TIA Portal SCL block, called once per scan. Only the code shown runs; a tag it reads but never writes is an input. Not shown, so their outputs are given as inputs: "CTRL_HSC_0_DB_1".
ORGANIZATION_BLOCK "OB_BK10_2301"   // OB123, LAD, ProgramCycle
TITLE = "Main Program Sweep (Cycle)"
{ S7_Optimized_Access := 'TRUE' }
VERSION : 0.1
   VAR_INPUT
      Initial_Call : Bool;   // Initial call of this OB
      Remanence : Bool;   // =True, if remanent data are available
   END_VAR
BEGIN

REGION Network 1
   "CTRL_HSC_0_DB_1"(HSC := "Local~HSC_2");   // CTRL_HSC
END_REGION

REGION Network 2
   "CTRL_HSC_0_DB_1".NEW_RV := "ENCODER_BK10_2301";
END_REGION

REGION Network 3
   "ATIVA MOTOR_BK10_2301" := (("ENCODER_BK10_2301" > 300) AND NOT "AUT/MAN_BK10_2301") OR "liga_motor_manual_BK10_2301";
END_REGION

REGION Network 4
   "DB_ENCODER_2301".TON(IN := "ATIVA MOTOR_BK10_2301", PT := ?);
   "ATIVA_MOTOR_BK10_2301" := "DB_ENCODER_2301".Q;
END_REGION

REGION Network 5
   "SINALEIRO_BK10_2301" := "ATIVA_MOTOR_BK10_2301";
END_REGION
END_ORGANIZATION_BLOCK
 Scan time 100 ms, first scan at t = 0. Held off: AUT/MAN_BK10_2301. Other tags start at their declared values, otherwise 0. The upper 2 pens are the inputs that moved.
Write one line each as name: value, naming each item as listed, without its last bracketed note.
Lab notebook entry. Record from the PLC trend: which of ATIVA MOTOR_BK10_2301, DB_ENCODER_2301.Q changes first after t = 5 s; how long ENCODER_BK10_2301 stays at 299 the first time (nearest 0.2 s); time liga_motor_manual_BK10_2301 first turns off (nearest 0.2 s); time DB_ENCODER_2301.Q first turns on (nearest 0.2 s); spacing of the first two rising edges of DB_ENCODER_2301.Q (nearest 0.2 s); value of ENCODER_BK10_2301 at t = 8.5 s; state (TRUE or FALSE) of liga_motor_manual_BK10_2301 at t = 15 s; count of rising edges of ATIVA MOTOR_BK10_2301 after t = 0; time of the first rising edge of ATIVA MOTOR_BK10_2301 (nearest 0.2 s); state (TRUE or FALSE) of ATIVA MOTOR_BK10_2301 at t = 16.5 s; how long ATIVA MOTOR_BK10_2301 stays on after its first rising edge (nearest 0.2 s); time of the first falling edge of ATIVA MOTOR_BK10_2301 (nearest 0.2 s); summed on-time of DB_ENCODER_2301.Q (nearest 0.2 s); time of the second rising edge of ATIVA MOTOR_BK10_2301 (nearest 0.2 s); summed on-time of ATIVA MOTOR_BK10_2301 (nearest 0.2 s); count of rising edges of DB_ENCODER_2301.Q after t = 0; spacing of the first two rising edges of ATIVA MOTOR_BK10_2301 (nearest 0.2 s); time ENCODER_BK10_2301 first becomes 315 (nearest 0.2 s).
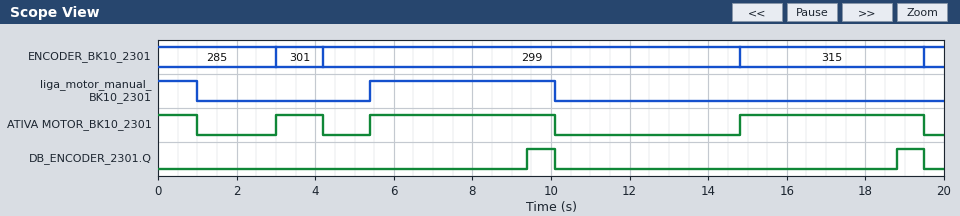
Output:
which of ATIVA MOTOR_BK10_2301, DB_ENCODER_2301.Q changes first after t = 5 s: ATIVA MOTOR_BK10_2301
how long ENCODER_BK10_2301 stays at 299 the first time: 10.6 s
time liga_motor_manual_BK10_2301 first turns off: 1.0 s
time DB_ENCODER_2301.Q first turns on: 9.4 s
spacing of the first two rising edges of DB_ENCODER_2301.Q: 9.4 s
value of ENCODER_BK10_2301 at t = 8.5 s: 299
state (TRUE or FALSE) of liga_motor_manual_BK10_2301 at t = 15 s: FALSE
count of rising edges of ATIVA MOTOR_BK10_2301 after t = 0: 3
time of the first rising edge of ATIVA MOTOR_BK10_2301: 3.0 s
state (TRUE or FALSE) of ATIVA MOTOR_BK10_2301 at t = 16.5 s: TRUE
how long ATIVA MOTOR_BK10_2301 stays on after its first rising edge: 1.2 s
time of the first falling edge of ATIVA MOTOR_BK10_2301: 1.0 s
summed on-time of DB_ENCODER_2301.Q: 1.4 s
time of the second rising edge of ATIVA MOTOR_BK10_2301: 5.4 s
summed on-time of ATIVA MOTOR_BK10_2301: 11.6 s
count of rising edges of DB_ENCODER_2301.Q after t = 0: 2
spacing of the first two rising edges of ATIVA MOTOR_BK10_2301: 2.4 s
time ENCODER_BK10_2301 first becomes 315: 14.8 s
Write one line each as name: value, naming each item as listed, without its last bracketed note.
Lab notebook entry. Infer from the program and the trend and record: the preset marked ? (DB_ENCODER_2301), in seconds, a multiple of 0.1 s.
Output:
the preset marked ? (DB_ENCODER_2301), in seconds, a multiple of 0.1 s: 4.0 s
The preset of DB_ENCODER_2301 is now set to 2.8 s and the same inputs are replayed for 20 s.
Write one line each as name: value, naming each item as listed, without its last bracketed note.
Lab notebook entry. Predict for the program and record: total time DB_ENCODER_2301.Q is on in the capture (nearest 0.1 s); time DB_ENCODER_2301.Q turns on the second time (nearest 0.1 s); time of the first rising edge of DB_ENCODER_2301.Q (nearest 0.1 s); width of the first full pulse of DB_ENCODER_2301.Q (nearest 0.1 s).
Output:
total time DB_ENCODER_2301.Q is on in the capture: 3.8 s
time DB_ENCODER_2301.Q turns on the second time: 17.6 s
time of the first rising edge of DB_ENCODER_2301.Q: 8.2 s
width of the first full pulse of DB_ENCODER_2301.Q: 1.9 s
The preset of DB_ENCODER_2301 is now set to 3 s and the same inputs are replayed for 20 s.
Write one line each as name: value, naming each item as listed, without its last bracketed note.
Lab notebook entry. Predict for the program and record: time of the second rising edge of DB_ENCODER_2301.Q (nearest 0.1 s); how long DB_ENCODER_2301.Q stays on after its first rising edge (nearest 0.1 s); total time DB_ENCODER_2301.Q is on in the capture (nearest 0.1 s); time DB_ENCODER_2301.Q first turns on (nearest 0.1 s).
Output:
time of the second rising edge of DB_ENCODER_2301.Q: 17.8 s
how long DB_ENCODER_2301.Q stays on after its first rising edge: 1.7 s
total time DB_ENCODER_2301.Q is on in the capture: 3.4 s
time DB_ENCODER_2301.Q first turns on: 8.4 s
